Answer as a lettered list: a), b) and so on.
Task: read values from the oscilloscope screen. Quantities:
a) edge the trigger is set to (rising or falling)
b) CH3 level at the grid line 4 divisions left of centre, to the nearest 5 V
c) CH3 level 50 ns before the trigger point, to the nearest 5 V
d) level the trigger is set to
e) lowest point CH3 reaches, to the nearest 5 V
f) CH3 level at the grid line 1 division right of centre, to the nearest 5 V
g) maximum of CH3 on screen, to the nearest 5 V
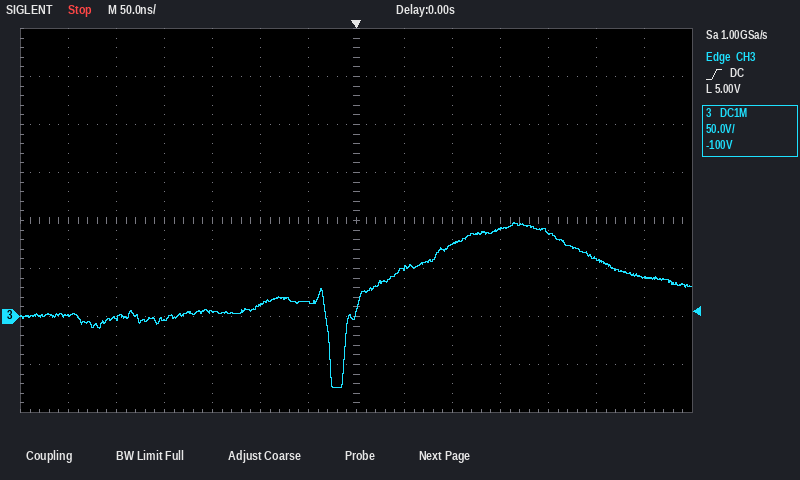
a) rising
b) -5 V
c) 15 V
d) 5.00 V
e) -75 V
f) 50 V
g) 100 V
